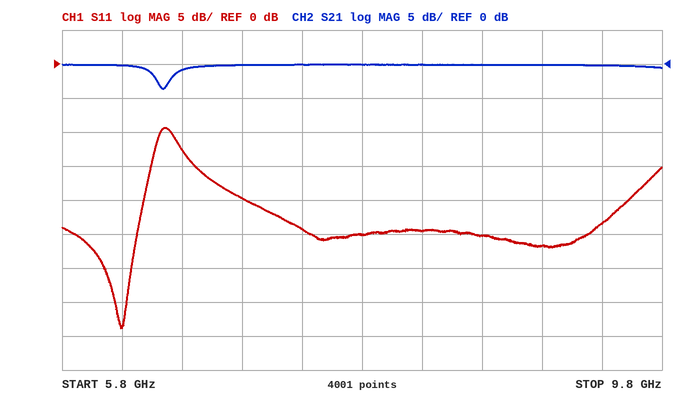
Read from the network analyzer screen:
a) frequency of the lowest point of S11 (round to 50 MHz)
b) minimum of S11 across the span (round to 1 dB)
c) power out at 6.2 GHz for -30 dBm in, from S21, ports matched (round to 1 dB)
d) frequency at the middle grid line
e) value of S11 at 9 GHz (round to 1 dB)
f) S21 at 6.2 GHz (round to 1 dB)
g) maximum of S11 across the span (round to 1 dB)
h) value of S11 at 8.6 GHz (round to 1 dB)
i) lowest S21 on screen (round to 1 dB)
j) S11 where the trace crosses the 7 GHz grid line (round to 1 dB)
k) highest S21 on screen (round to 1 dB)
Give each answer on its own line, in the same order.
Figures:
6.20 GHz
-39 dB
-30 dBm
7.8 GHz
-27 dB
0 dB
-9 dB
-25 dB
-4 dB
-20 dB
0 dB
